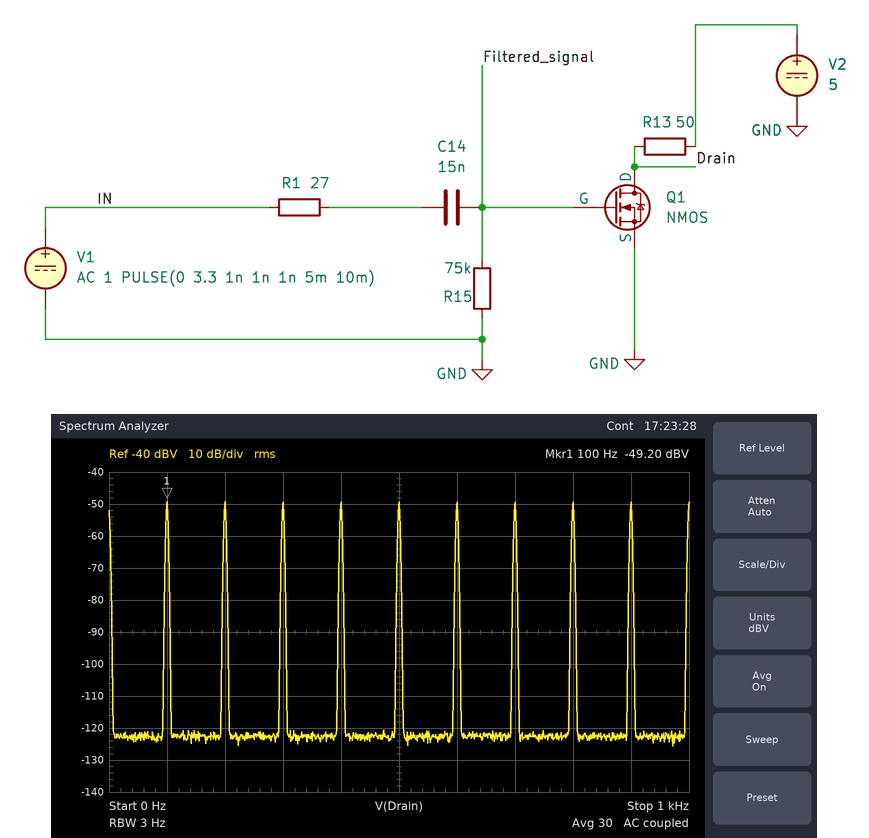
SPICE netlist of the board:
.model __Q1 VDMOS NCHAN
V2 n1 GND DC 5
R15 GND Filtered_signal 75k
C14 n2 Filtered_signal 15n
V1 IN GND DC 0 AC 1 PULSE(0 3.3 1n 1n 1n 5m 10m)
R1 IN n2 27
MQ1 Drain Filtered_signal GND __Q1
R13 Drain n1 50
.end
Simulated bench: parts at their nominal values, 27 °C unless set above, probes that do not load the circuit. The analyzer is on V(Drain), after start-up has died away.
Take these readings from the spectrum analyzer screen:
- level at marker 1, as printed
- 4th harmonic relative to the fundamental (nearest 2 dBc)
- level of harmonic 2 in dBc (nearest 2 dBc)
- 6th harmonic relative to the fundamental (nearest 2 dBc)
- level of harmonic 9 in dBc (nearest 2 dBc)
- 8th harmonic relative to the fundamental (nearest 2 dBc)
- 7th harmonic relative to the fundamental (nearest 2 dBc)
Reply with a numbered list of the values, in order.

1. -49.20 dBV
2. 0 dBc
3. 0 dBc
4. 0 dBc
5. 0 dBc
6. 0 dBc
7. 0 dBc
